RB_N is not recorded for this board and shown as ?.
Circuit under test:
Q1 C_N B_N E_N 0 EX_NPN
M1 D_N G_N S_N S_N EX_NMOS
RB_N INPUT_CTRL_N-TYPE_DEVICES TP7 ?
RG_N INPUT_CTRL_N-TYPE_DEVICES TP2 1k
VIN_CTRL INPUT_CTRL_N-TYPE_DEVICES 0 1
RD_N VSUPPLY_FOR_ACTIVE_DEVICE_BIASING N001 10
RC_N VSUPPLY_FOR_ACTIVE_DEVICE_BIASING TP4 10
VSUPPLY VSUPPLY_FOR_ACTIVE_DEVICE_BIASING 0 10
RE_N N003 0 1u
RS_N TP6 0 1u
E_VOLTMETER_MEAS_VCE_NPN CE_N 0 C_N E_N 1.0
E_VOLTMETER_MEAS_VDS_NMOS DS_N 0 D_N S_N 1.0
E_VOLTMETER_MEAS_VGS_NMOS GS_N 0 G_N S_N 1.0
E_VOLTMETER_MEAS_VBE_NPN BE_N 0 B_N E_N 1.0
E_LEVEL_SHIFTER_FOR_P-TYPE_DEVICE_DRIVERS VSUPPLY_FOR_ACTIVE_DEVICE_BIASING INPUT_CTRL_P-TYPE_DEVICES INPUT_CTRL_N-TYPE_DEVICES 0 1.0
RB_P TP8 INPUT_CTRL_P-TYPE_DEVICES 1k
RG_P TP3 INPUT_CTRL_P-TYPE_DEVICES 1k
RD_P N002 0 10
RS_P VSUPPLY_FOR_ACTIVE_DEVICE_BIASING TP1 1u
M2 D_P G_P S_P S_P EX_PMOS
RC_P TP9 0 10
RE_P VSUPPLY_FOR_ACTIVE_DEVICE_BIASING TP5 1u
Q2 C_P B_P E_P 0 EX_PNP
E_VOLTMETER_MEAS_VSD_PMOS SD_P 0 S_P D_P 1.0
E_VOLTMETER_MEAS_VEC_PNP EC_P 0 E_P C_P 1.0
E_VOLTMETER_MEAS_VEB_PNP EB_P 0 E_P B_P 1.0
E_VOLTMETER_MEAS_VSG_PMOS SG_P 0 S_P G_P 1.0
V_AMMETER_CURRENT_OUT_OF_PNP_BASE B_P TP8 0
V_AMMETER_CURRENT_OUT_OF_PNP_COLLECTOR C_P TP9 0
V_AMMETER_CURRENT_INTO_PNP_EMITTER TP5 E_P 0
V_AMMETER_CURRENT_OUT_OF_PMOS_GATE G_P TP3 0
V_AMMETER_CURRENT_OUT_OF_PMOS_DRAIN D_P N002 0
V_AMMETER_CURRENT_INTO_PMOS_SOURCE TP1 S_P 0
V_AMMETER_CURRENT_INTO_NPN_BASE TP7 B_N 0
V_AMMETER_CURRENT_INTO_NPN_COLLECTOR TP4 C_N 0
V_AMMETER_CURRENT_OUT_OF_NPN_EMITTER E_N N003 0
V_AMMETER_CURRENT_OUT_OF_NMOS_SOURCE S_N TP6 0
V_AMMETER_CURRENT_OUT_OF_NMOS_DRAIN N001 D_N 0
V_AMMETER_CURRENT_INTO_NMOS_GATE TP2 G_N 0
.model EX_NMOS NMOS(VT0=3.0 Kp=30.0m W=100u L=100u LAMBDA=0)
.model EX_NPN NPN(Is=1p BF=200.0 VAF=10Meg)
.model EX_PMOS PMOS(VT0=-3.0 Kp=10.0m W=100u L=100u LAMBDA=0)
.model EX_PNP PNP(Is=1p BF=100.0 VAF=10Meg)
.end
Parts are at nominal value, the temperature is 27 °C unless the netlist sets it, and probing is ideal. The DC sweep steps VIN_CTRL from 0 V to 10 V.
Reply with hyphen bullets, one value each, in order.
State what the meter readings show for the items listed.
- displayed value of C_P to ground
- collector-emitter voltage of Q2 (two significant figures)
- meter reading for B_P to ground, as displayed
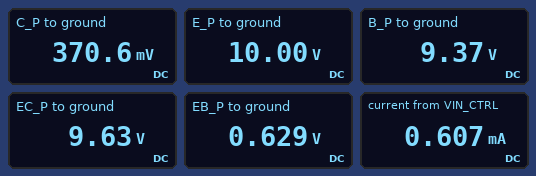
- 370.6 mV
- -9.6 V
- 9.37 V
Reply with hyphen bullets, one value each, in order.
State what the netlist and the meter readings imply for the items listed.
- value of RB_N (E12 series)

- 560 Ω
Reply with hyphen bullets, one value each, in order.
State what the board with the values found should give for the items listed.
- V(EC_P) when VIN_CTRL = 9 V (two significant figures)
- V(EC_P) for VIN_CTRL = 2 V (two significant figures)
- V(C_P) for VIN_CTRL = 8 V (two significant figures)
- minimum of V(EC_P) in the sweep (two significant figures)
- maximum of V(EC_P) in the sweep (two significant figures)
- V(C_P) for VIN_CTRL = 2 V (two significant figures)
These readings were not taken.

- 1.7 V
- 8.7 V
- 7.3 V
- 710 mV
- 10 V
- 1.3 V
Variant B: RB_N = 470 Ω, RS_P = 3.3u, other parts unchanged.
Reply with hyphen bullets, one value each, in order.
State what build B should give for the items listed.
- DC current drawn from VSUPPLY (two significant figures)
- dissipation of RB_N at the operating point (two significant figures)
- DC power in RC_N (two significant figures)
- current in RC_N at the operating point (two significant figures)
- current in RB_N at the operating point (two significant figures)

- 180 mA
- 240 µW
- 200 mW
- 140 mA
- 710 µA
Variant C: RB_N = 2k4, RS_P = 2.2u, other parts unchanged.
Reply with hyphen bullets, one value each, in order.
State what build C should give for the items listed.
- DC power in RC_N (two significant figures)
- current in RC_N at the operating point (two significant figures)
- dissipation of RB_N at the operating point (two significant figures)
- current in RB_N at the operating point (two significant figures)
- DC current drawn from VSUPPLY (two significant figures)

- 9.8 mW
- 31 mA
- 59 µW
- 160 µA
- 68 mA
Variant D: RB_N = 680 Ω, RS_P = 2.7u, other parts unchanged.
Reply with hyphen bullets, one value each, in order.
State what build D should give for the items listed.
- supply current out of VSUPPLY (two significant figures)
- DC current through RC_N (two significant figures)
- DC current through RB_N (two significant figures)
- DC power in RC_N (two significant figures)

- 140 mA
- 100 mA
- 510 µA
- 100 mW
